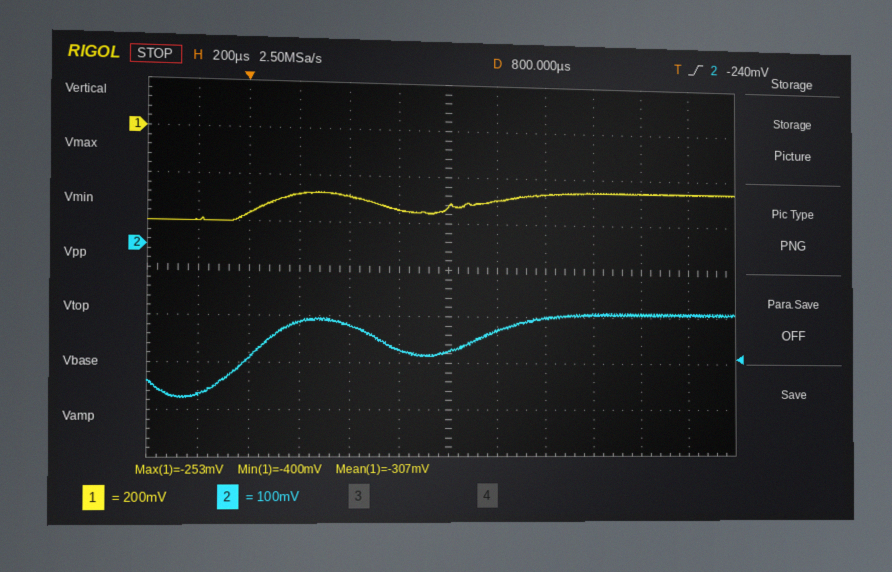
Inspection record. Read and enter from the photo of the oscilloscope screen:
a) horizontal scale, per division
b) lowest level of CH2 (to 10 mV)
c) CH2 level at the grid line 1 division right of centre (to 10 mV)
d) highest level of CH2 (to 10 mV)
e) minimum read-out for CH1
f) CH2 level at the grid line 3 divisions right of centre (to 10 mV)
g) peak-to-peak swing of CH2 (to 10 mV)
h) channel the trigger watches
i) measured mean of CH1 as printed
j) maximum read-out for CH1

200 µs
-320 mV
-180 mV
-140 mV
-400 mV
-140 mV
180 mV
CH2
-307 mV
-253 mV
